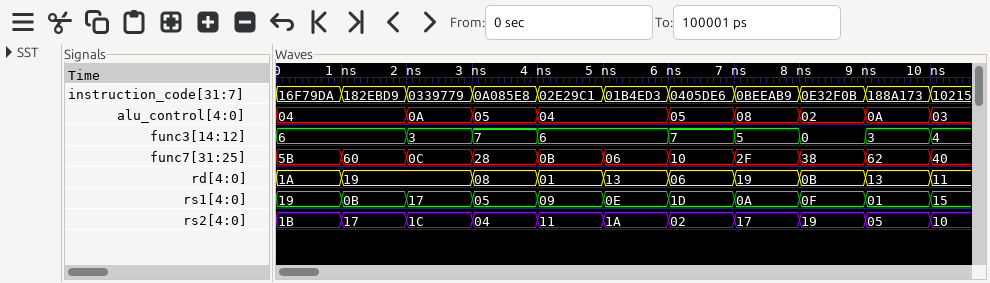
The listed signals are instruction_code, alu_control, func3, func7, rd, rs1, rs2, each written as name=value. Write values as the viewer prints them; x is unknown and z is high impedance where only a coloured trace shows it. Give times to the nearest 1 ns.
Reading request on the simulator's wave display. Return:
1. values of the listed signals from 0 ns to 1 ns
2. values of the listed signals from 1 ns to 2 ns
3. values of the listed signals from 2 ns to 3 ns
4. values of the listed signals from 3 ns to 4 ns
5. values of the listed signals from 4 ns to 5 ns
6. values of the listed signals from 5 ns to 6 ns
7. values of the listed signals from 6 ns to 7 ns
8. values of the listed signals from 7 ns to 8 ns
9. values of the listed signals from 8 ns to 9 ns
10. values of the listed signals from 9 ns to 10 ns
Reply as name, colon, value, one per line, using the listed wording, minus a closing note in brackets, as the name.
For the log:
values of the listed signals from 0 ns to 1 ns: instruction_code=16F79DA, alu_control=04, func3=6, func7=5B, rd=1A, rs1=19, rs2=1B
values of the listed signals from 1 ns to 2 ns: instruction_code=182EBD9, alu_control=04, func3=6, func7=60, rd=19, rs1=0B, rs2=17
values of the listed signals from 2 ns to 3 ns: instruction_code=0339779, alu_control=0A, func3=3, func7=0C, rd=19, rs1=17, rs2=1C
values of the listed signals from 3 ns to 4 ns: instruction_code=0A085E8, alu_control=05, func3=7, func7=28, rd=08, rs1=05, rs2=04
values of the listed signals from 4 ns to 5 ns: instruction_code=02E29C1, alu_control=04, func3=6, func7=0B, rd=01, rs1=09, rs2=11
values of the listed signals from 5 ns to 6 ns: instruction_code=01B4ED3, alu_control=04, func3=6, func7=06, rd=13, rs1=0E, rs2=1A
values of the listed signals from 6 ns to 7 ns: instruction_code=0405DE6, alu_control=05, func3=7, func7=10, rd=06, rs1=1D, rs2=02
values of the listed signals from 7 ns to 8 ns: instruction_code=0BEEAB9, alu_control=08, func3=5, func7=2F, rd=19, rs1=0A, rs2=17
values of the listed signals from 8 ns to 9 ns: instruction_code=0E32F0B, alu_control=02, func3=0, func7=38, rd=0B, rs1=0F, rs2=19
values of the listed signals from 9 ns to 10 ns: instruction_code=188A173, alu_control=0A, func3=3, func7=62, rd=13, rs1=01, rs2=05
